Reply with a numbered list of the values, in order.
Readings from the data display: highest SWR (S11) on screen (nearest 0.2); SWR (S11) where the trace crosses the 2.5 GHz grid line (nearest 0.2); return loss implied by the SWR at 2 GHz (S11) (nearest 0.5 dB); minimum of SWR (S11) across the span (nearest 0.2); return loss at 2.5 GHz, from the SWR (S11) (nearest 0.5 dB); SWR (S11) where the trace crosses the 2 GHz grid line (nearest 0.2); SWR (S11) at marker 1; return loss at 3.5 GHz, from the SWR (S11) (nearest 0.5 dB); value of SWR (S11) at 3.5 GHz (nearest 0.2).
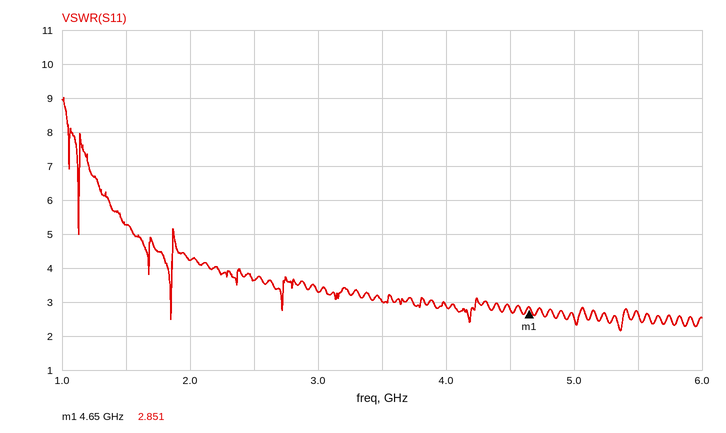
1. 9.0
2. 3.6
3. 4.0 dB
4. 2.2
5. 5.0 dB
6. 4.2
7. 2.851
8. 6.0 dB
9. 3.0
